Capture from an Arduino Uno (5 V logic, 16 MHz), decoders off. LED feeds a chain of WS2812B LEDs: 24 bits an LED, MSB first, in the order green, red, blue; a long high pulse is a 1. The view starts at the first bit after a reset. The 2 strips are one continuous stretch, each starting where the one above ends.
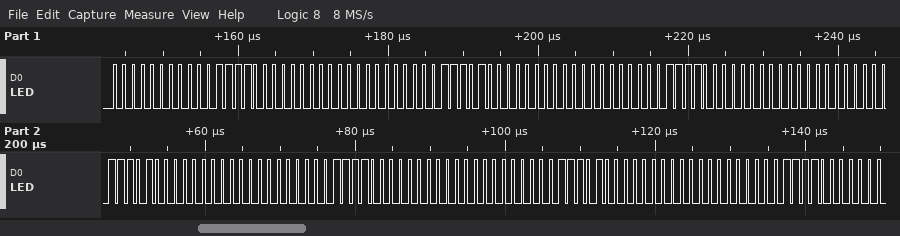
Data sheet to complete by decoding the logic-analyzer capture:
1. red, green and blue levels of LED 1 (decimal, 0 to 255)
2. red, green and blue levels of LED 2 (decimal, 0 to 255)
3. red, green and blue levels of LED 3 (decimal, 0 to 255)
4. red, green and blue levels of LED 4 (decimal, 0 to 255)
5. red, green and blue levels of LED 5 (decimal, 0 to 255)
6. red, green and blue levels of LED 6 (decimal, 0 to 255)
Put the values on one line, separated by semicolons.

30, 0, 0; 29, 0, 0; 30, 0, 0; 29, 0, 0; 30, 0, 0; 29, 0, 0
